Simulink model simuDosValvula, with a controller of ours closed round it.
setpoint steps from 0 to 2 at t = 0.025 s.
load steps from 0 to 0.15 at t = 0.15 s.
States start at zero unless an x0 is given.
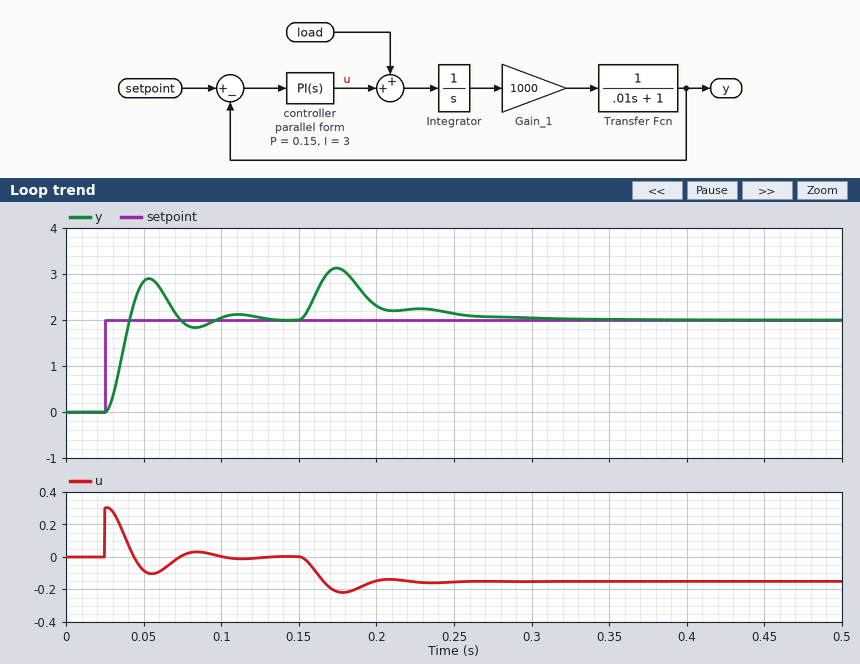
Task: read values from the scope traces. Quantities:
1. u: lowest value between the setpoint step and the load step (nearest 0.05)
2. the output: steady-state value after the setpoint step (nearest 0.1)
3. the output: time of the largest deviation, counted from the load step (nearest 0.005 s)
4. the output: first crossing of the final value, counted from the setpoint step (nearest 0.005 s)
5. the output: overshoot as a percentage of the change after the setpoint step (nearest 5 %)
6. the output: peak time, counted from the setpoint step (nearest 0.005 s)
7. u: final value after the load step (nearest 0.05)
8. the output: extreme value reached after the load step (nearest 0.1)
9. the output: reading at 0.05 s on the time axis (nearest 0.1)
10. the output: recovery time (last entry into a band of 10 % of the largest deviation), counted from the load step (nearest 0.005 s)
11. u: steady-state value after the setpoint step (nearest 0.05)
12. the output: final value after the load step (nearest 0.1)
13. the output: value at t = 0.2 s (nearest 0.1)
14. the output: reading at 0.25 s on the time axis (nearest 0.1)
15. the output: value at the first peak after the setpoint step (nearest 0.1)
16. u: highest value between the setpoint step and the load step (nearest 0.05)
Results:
-0.10
2.0
0.025 s
0.015 s
45 %
0.030 s
-0.15
3.1
2.8
0.105 s
0.00
2.0
2.3
2.1
2.9
0.30
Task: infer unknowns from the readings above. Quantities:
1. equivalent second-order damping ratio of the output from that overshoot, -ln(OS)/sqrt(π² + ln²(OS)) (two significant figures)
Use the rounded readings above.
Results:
0.25
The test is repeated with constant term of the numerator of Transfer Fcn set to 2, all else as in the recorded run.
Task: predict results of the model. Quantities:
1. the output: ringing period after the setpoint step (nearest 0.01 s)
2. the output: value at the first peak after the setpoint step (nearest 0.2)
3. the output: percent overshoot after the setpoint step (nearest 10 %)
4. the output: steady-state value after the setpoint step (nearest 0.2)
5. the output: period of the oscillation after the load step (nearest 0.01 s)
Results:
0.04 s
3.0
50 %
2.0
0.04 s
